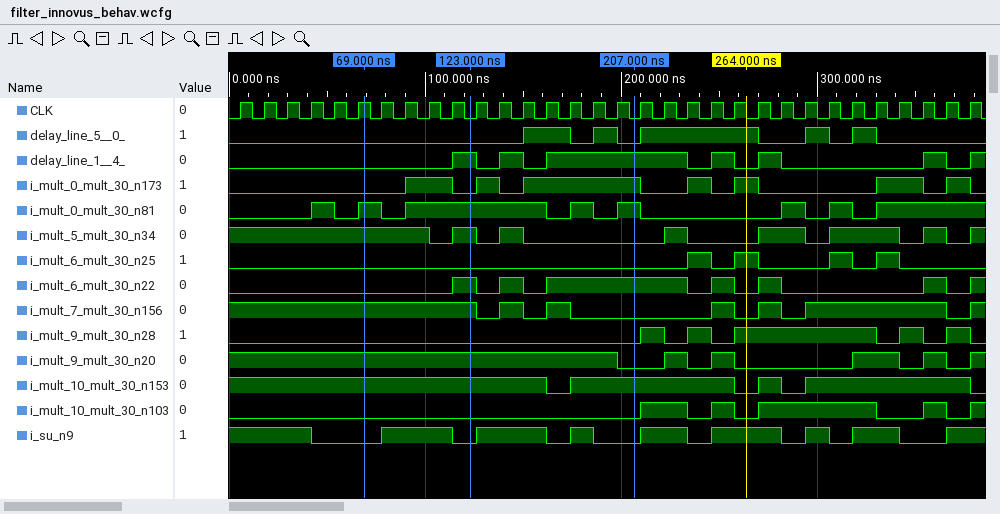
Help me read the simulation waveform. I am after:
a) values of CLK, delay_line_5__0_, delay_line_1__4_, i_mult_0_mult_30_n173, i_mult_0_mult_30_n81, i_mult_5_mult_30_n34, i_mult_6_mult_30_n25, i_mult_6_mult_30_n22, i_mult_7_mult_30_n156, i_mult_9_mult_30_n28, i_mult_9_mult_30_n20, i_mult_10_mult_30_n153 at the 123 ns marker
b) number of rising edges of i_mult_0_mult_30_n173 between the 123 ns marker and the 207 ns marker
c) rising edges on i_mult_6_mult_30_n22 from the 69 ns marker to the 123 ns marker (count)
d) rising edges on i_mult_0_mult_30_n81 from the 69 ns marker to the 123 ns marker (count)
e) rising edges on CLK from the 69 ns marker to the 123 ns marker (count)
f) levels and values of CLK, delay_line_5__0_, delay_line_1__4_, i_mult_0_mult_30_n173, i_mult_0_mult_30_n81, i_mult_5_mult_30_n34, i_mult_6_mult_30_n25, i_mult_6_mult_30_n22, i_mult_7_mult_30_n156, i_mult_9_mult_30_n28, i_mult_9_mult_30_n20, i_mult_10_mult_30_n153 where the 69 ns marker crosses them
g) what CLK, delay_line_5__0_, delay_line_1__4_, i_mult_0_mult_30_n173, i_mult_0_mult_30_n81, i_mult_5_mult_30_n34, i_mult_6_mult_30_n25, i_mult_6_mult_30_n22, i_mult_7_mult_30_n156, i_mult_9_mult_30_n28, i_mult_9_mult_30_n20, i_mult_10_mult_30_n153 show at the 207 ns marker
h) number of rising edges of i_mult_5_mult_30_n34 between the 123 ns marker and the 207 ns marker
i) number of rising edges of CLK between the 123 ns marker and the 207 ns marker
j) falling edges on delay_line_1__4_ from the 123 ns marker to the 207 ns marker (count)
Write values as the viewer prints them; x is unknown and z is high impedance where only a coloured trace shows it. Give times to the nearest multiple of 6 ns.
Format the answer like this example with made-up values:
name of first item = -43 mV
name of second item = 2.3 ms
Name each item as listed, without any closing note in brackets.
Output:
values of CLK, delay_line_5__0_, delay_line_1__4_, i_mult_0_mult_30_n173, i_mult_0_mult_30_n81, i_mult_5_mult_30_n34, i_mult_6_mult_30_n25, i_mult_6_mult_30_n22, i_mult_7_mult_30_n156, i_mult_9_mult_30_n28, i_mult_9_mult_30_n20, i_mult_10_mult_30_n153 at the 123 ns marker = CLK=0, delay_line_5__0_=0, delay_line_1__4_=1, i_mult_0_mult_30_n173=0, i_mult_0_mult_30_n81=1, i_mult_5_mult_30_n34=1, i_mult_6_mult_30_n25=0, i_mult_6_mult_30_n22=1, i_mult_7_mult_30_n156=1, i_mult_9_mult_30_n28=0, i_mult_9_mult_30_n20=1, i_mult_10_mult_30_n153=1
number of rising edges of i_mult_0_mult_30_n173 between the 123 ns marker and the 207 ns marker = 2
rising edges on i_mult_6_mult_30_n22 from the 69 ns marker to the 123 ns marker = 1
rising edges on i_mult_0_mult_30_n81 from the 69 ns marker to the 123 ns marker = 1
rising edges on CLK from the 69 ns marker to the 123 ns marker = 4
levels and values of CLK, delay_line_5__0_, delay_line_1__4_, i_mult_0_mult_30_n173, i_mult_0_mult_30_n81, i_mult_5_mult_30_n34, i_mult_6_mult_30_n25, i_mult_6_mult_30_n22, i_mult_7_mult_30_n156, i_mult_9_mult_30_n28, i_mult_9_mult_30_n20, i_mult_10_mult_30_n153 where the 69 ns marker crosses them = CLK=1, delay_line_5__0_=0, delay_line_1__4_=0, i_mult_0_mult_30_n173=0, i_mult_0_mult_30_n81=1, i_mult_5_mult_30_n34=1, i_mult_6_mult_30_n25=0, i_mult_6_mult_30_n22=0, i_mult_7_mult_30_n156=1, i_mult_9_mult_30_n28=0, i_mult_9_mult_30_n20=1, i_mult_10_mult_30_n153=1
what CLK, delay_line_5__0_, delay_line_1__4_, i_mult_0_mult_30_n173, i_mult_0_mult_30_n81, i_mult_5_mult_30_n34, i_mult_6_mult_30_n25, i_mult_6_mult_30_n22, i_mult_7_mult_30_n156, i_mult_9_mult_30_n28, i_mult_9_mult_30_n20, i_mult_10_mult_30_n153 show at the 207 ns marker = CLK=0, delay_line_5__0_=0, delay_line_1__4_=1, i_mult_0_mult_30_n173=1, i_mult_0_mult_30_n81=1, i_mult_5_mult_30_n34=0, i_mult_6_mult_30_n25=0, i_mult_6_mult_30_n22=1, i_mult_7_mult_30_n156=0, i_mult_9_mult_30_n28=0, i_mult_9_mult_30_n20=0, i_mult_10_mult_30_n153=1
number of rising edges of i_mult_5_mult_30_n34 between the 123 ns marker and the 207 ns marker = 1
number of rising edges of CLK between the 123 ns marker and the 207 ns marker = 7
falling edges on delay_line_1__4_ from the 123 ns marker to the 207 ns marker = 2
